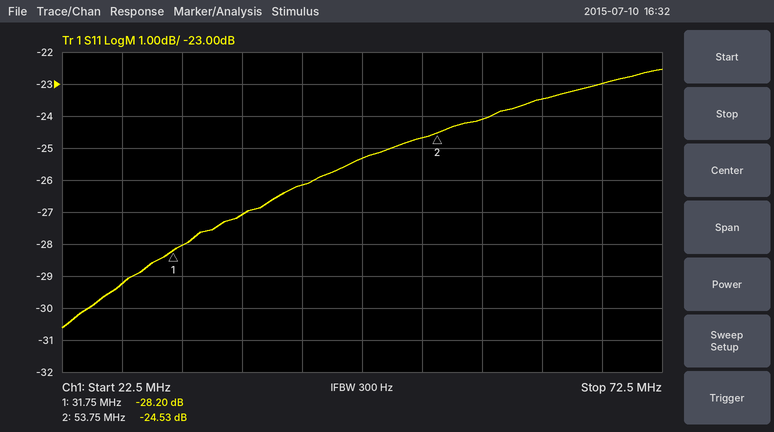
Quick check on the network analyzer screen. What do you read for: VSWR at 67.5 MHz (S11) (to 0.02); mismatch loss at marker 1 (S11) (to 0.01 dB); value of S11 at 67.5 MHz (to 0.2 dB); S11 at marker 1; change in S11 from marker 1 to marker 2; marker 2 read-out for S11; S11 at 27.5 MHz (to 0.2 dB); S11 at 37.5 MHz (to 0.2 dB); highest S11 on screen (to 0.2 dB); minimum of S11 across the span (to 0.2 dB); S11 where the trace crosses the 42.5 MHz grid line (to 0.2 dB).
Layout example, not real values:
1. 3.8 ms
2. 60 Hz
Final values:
1. 1.16
2. 0.01 dB
3. -23.0 dB
4. -28.20 dB
5. 3.67 dB
6. -24.53 dB
7. -29.2 dB
8. -27.0 dB
9. -22.6 dB
10. -30.6 dB
11. -26.2 dB
